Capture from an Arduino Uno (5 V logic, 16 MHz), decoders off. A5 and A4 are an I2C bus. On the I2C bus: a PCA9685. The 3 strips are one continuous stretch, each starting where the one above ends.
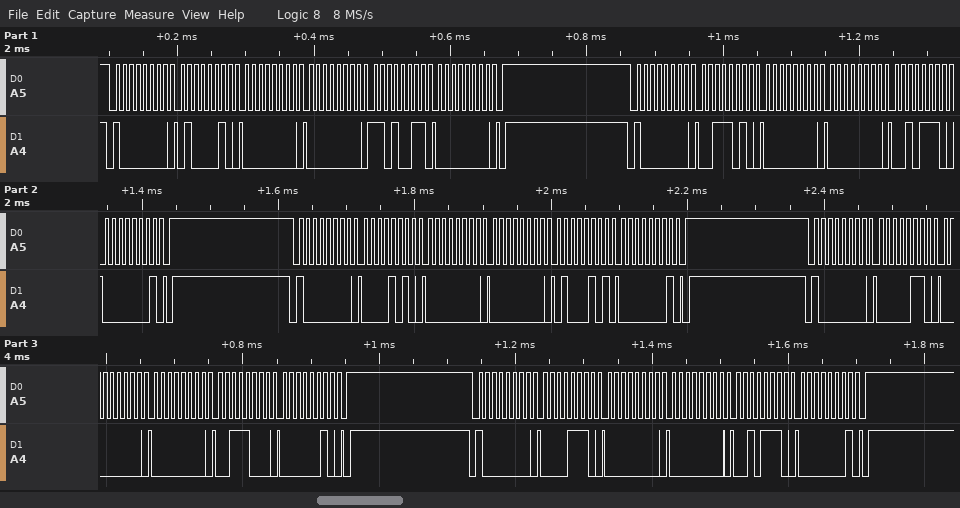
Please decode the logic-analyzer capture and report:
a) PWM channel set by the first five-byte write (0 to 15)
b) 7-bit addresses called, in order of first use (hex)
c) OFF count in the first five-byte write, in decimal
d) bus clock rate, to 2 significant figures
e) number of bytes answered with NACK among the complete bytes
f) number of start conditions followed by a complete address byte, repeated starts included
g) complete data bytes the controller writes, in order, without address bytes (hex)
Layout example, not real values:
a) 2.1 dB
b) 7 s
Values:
a) 15
b) 0x40
c) 211
d) 100 kHz
e) 0
f) 5
g) 42 00 00 D3 00 3A 00 00 2E 01 0A 00 00 45 01 06 00 00 38 02 0E 00 00 2E 01
